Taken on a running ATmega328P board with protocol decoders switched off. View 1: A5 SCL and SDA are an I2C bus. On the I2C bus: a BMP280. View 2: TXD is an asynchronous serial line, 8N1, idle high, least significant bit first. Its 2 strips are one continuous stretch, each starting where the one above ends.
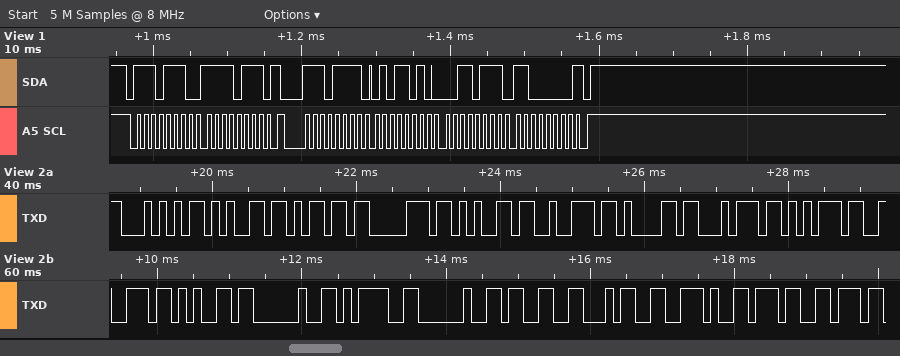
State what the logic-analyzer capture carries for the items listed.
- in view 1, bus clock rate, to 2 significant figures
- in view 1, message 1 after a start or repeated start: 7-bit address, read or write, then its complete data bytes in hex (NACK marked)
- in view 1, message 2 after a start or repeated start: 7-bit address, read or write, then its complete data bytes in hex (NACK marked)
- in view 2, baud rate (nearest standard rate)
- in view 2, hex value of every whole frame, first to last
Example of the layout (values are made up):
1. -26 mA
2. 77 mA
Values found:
1. 100 kHz
2. 0x77 write: F7
3. 0x77 read: 5A 37 C0 NACK
4. 9600 baud
5. 54 65 6D 70 65 72 61 74 75 72 65 20 3D 20 33 34 2E 37
